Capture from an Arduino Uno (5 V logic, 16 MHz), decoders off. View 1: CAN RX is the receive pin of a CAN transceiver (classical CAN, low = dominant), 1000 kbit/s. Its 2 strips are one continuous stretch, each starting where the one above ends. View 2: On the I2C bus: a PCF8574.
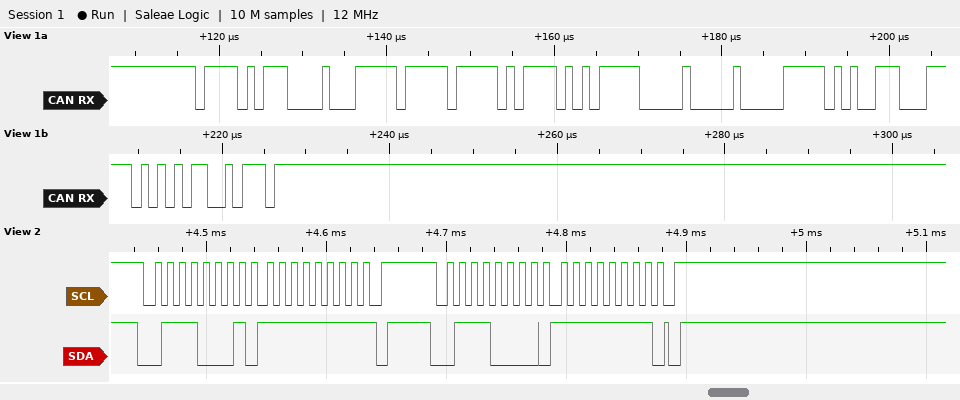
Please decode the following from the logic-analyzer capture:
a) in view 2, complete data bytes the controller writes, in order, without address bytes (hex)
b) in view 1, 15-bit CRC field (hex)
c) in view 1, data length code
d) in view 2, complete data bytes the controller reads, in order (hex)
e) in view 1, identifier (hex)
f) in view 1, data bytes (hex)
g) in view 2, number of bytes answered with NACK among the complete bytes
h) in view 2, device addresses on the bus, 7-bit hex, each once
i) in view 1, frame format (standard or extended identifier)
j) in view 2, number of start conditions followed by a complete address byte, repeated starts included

FF
0x6ACB
8
FF
0x7AE
FF FF 7A BE 00 07 D3 8F
1
0x38
standard
2
